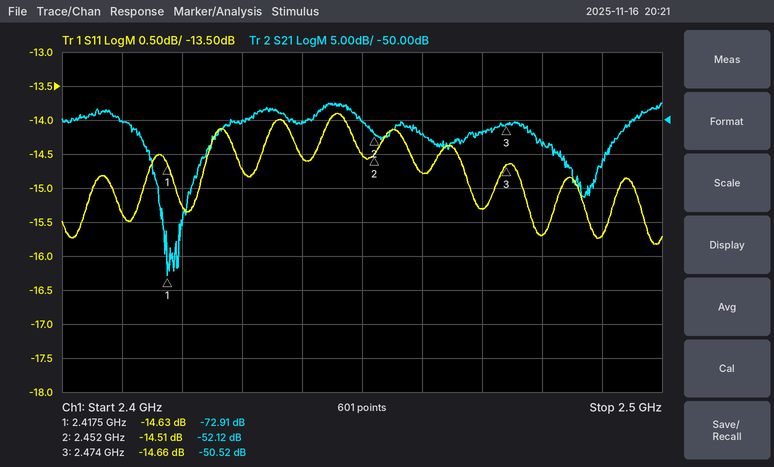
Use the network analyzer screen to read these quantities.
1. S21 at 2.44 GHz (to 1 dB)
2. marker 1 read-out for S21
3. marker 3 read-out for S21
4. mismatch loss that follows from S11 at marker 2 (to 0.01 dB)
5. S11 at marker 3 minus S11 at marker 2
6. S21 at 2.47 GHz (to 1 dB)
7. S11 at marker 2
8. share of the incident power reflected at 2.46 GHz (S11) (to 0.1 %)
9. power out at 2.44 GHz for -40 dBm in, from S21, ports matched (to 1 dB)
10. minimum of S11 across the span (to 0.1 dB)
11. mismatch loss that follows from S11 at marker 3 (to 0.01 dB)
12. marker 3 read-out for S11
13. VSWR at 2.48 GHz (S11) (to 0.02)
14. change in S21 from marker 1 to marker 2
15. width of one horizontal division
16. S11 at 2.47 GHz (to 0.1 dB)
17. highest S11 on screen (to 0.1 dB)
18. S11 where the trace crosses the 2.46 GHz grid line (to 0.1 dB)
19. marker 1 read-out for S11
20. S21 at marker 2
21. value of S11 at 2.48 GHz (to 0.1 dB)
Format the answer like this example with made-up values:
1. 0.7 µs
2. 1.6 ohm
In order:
1. -50 dB
2. -72.91 dB
3. -50.52 dB
4. 0.16 dB
5. -0.15 dB
6. -52 dB
7. -14.51 dB
8. 3.3 %
9. -90 dBm
10. -15.8 dB
11. 0.15 dB
12. -14.66 dB
13. 1.40
14. 20.79 dB
15. 10 MHz
16. -15.3 dB
17. -13.9 dB
18. -14.8 dB
19. -14.63 dB
20. -52.12 dB
21. -15.7 dB
